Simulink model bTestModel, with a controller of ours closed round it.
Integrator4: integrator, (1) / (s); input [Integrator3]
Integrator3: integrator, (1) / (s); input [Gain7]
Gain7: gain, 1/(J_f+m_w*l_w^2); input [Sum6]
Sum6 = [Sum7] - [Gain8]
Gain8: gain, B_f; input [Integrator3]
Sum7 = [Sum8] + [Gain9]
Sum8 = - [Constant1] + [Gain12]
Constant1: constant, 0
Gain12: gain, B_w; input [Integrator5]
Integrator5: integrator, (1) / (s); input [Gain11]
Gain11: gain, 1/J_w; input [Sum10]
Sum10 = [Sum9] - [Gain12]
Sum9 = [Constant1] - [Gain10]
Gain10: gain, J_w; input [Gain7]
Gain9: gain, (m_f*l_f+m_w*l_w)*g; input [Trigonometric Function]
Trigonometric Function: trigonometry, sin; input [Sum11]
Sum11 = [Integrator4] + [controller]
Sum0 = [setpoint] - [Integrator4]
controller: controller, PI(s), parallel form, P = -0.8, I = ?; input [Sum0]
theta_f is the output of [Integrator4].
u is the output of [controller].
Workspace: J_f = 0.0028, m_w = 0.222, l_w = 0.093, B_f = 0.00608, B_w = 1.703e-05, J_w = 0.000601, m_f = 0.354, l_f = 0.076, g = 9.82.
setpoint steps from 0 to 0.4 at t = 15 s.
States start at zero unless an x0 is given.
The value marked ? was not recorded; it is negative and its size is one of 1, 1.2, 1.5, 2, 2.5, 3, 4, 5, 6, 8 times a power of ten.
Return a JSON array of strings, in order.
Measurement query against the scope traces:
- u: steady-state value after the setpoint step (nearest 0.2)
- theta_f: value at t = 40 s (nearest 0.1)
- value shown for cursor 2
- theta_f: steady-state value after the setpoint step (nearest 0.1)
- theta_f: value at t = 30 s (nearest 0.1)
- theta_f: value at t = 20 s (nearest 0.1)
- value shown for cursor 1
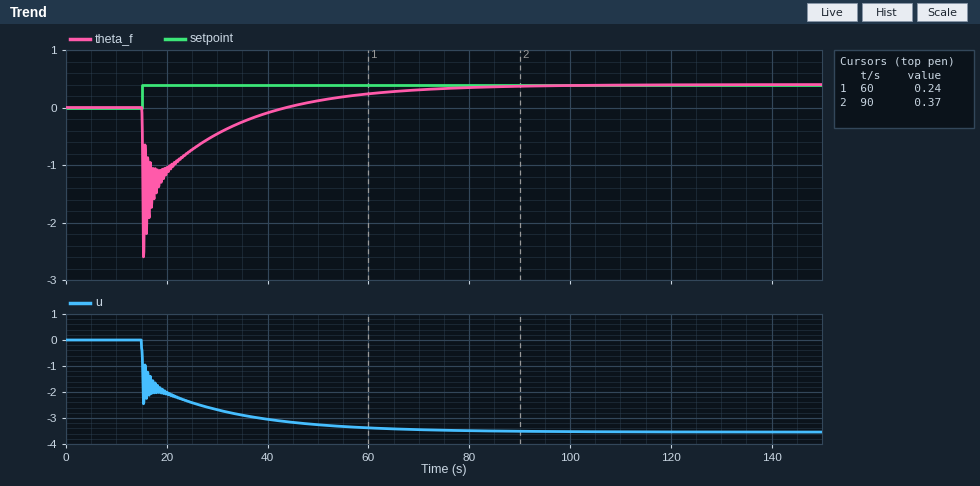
["-3.6", "-0.1", "0.37", "0.4", "-0.5", "-1.1", "0.24"]
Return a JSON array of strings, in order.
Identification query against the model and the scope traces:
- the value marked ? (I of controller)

["-0.1"]
